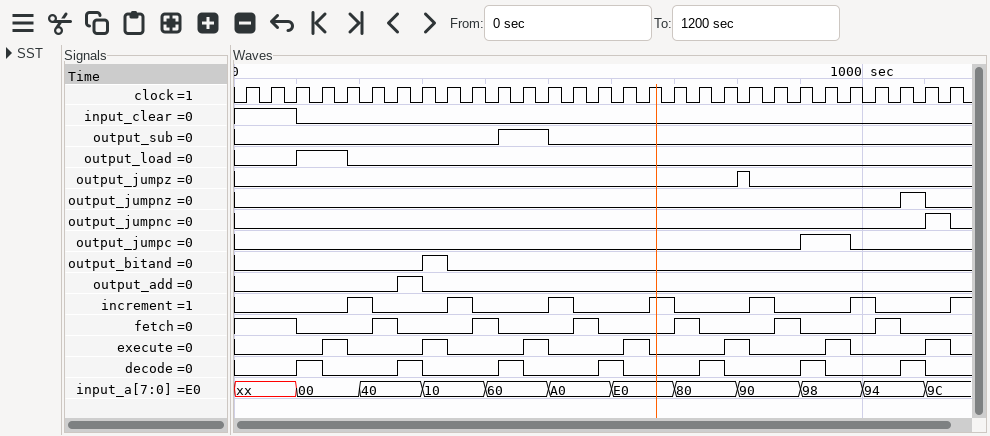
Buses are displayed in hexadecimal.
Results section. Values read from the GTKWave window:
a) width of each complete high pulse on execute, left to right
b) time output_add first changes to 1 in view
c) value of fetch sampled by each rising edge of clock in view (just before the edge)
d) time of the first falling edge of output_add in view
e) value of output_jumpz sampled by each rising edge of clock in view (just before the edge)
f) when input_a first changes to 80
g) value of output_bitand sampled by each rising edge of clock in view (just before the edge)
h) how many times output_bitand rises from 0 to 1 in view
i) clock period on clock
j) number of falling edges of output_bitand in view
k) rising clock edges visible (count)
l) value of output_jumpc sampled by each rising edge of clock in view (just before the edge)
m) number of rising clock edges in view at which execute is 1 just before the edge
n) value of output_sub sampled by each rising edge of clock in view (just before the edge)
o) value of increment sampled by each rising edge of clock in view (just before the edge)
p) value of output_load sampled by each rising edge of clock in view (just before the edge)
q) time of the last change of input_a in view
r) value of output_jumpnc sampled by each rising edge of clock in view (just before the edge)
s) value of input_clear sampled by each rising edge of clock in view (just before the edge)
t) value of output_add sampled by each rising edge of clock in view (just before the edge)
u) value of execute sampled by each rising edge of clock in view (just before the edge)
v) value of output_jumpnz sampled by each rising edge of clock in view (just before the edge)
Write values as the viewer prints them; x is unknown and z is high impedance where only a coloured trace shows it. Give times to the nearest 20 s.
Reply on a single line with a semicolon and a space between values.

40 s, 40 s, 40 s, 40 s, 40 s, 40 s, 40 s; 260 s; 1 1 1 0 0 0 1 0 0 0 1 0 0 0 1 0 0 0 1 0 0 0 1 0 0 0 1 0 0; 300 s; 0 0 0 0 0 0 0 0 0 0 0 0 0 0 0 0 0 0 0 0 1 0 0 0 0 0 0 0 0; 700 s; 0 0 0 0 0 0 0 0 1 0 0 0 0 0 0 0 0 0 0 0 0 0 0 0 0 0 0 0 0; 1; 40 s; 1; 29; 0 0 0 0 0 0 0 0 0 0 0 0 0 0 0 0 0 0 0 0 0 0 0 1 1 0 0 0 0; 7; 0 0 0 0 0 0 0 0 0 0 0 1 1 0 0 0 0 0 0 0 0 0 0 0 0 0 0 0 0; 0 0 0 0 0 1 0 0 0 1 0 0 0 1 0 0 0 1 0 0 0 1 0 0 0 1 0 0 0; 0 0 0 1 1 0 0 0 0 0 0 0 0 0 0 0 0 0 0 0 0 0 0 0 0 0 0 0 0; 1100 s; 0 0 0 0 0 0 0 0 0 0 0 0 0 0 0 0 0 0 0 0 0 0 0 0 0 0 0 0 1; 1 1 1 0 0 0 0 0 0 0 0 0 0 0 0 0 0 0 0 0 0 0 0 0 0 0 0 0 0; 0 0 0 0 0 0 0 1 0 0 0 0 0 0 0 0 0 0 0 0 0 0 0 0 0 0 0 0 0; 0 0 0 0 1 0 0 0 1 0 0 0 1 0 0 0 1 0 0 0 1 0 0 0 1 0 0 0 1; 0 0 0 0 0 0 0 0 0 0 0 0 0 0 0 0 0 0 0 0 0 0 0 0 0 0 0 1 0
